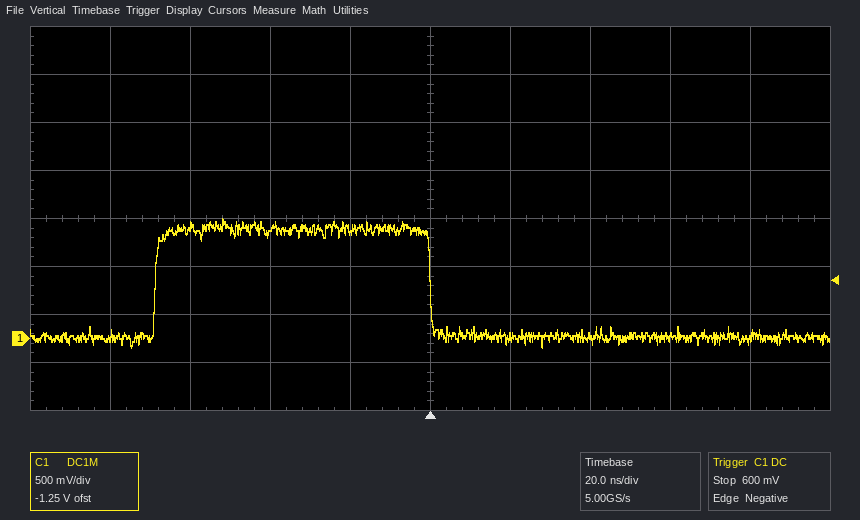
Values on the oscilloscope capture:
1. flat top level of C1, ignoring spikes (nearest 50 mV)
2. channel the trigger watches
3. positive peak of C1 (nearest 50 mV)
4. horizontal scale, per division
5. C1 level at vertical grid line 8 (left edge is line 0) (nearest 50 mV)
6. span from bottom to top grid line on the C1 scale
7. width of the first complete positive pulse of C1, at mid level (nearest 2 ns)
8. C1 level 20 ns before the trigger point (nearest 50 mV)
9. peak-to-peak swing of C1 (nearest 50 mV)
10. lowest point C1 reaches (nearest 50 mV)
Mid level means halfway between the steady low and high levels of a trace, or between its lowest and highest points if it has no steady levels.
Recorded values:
1.15 V
C1
1.25 V
20 ns
0 mV
4 V
68 ns
1.15 V
1.35 V
-100 mV
